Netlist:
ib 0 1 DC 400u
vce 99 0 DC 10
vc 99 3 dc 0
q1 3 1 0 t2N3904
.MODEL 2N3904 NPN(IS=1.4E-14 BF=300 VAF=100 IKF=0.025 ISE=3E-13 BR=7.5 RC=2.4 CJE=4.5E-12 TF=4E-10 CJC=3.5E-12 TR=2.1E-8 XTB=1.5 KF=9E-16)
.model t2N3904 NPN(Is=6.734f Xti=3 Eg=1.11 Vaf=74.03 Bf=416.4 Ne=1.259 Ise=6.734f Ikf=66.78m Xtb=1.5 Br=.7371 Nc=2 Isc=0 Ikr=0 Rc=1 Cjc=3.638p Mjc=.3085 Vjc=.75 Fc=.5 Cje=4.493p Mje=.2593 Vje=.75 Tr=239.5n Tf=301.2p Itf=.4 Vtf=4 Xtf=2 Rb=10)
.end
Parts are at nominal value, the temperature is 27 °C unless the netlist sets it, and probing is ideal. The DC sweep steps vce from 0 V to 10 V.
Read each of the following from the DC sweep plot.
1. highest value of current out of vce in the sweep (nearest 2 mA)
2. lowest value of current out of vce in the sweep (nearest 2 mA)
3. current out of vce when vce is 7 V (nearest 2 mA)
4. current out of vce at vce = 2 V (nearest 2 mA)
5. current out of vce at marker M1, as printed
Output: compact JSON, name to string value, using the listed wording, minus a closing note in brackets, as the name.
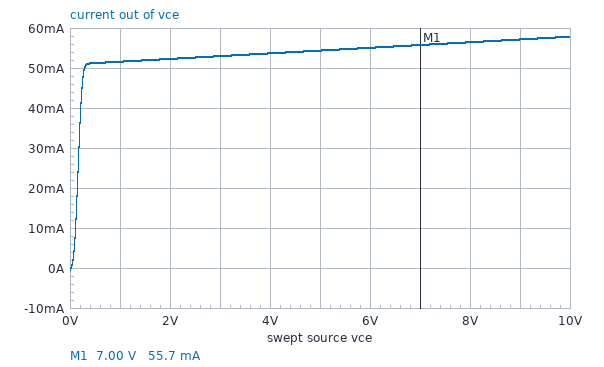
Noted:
{"highest value of current out of vce in the sweep": "58 mA", "lowest value of current out of vce in the sweep": "0 A", "current out of vce when vce is 7 V": "56 mA", "current out of vce at vce = 2 V": "52 mA", "current out of vce at marker M1, as printed": "55.7 mA"}
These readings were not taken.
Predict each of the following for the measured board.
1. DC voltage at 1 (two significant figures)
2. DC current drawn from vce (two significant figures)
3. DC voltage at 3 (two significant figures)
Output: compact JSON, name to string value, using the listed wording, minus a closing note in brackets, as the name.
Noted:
{"DC voltage at 1": "790 mV", "DC current drawn from vce": "58 mA", "DC voltage at 3": "10 V"}
